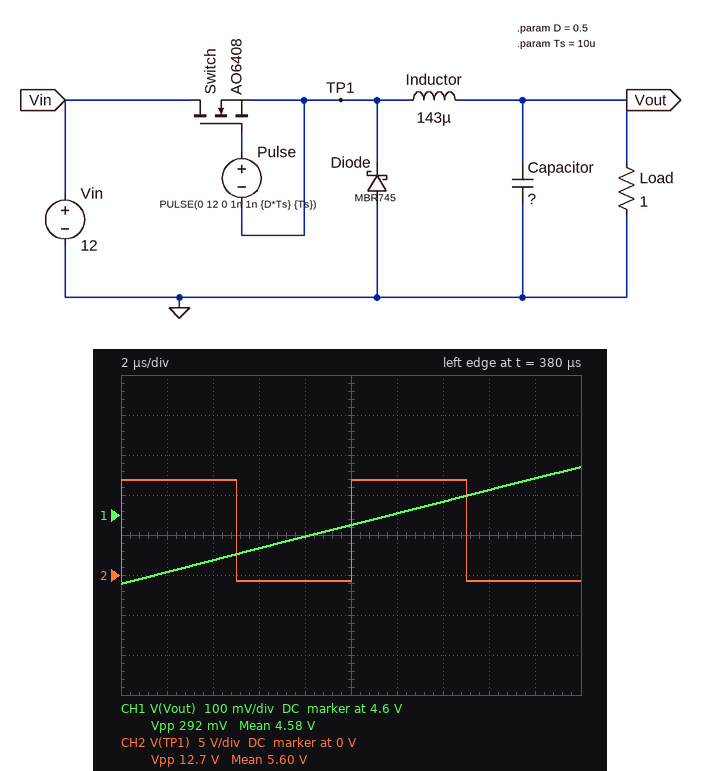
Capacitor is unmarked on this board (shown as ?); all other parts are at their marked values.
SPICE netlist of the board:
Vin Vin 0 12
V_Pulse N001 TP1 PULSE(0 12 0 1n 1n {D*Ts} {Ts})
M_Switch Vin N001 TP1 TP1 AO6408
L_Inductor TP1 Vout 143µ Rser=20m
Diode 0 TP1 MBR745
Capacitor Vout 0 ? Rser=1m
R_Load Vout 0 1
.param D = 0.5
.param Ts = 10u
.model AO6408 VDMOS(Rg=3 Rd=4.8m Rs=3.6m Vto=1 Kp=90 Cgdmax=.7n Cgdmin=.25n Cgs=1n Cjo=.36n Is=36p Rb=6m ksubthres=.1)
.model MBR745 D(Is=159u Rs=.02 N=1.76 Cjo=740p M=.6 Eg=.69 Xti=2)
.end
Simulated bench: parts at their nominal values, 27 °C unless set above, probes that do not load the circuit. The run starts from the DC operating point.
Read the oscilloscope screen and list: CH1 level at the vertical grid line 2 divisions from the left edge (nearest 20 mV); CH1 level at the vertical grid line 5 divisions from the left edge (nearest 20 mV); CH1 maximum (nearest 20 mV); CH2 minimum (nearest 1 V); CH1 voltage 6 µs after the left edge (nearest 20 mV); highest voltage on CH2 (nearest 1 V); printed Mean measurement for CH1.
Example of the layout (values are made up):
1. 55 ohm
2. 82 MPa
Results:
1. 4.48 V
2. 4.58 V
3. 4.72 V
4. -1 V
5. 4.52 V
6. 12 V
7. 4.58 V
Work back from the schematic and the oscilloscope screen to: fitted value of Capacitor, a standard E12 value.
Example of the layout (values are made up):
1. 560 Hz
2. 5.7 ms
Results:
1. 390 µF
